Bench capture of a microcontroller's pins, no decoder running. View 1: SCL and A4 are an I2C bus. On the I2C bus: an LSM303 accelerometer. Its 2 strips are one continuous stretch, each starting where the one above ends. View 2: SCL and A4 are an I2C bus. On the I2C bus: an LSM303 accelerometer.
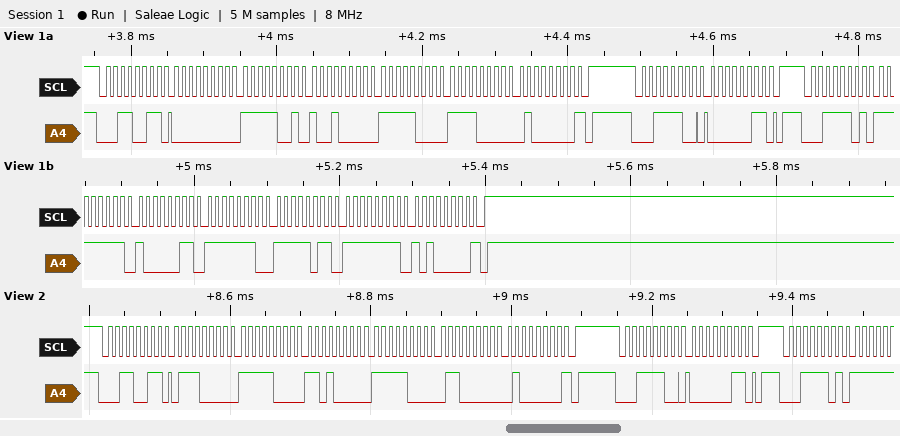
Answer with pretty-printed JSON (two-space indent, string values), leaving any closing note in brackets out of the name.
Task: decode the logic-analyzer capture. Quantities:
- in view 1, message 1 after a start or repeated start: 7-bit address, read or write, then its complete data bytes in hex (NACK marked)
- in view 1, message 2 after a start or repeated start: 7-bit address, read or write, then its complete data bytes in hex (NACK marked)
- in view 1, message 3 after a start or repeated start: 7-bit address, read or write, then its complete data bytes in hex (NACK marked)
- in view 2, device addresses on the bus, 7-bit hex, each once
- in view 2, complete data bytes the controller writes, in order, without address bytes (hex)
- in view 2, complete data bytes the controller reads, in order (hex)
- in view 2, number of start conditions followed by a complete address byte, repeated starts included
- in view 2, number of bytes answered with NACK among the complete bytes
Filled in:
{
  "in view 1, message 1 after a start or repeated start: 7-bit address, read or write, then its complete data bytes in hex": "0x19 read: 00 F9 90 F8 F0 40 NACK",
  "in view 1, message 2 after a start or repeated start: 7-bit address, read or write, then its complete data bytes in hex": "0x1E write: 03",
  "in view 1, message 3 after a start or repeated start: 7-bit address, read or write, then its complete data bytes in hex": "0x1E read: FF 83 FE FB FF A0 NACK",
  "in view 2, device addresses on the bus, 7-bit hex, each once": "0x19 0x1E",
  "in view 2, complete data bytes the controller writes, in order, without address bytes": "03",
  "in view 2, complete data bytes the controller reads, in order": "70 F8 D0 F8 60 40",
  "in view 2, number of start conditions followed by a complete address byte, repeated starts included": "3",
  "in view 2, number of bytes answered with NACK among the complete bytes": "1"
}
